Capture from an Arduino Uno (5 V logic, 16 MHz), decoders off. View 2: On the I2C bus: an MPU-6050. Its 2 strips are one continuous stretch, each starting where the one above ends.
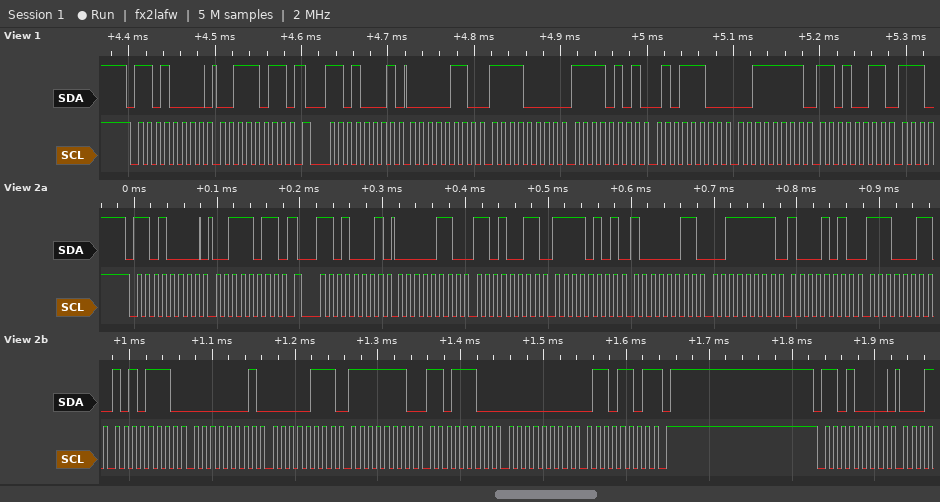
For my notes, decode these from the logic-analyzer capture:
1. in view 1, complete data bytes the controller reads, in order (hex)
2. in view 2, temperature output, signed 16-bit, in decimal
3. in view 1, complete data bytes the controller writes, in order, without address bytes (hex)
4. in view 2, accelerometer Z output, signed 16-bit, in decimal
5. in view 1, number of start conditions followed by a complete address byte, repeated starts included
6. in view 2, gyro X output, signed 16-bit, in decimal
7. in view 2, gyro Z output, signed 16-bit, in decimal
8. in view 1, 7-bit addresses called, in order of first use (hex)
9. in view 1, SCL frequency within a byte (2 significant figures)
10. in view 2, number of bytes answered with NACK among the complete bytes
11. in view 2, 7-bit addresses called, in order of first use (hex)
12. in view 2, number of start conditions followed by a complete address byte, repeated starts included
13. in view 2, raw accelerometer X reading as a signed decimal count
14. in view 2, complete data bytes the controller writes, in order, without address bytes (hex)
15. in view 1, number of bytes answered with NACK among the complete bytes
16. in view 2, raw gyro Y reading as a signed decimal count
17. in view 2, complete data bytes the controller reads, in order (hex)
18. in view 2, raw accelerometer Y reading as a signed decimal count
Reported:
06 F0 F5 5C 3F D3
-7250
3B
16266
2
263
109
0x68
100 kHz
1
0x68
3
1747
3B
0
-292
06 D3 F5 83 3F 8A E3 AE 01 07 FE DC 00 6D
-2685
